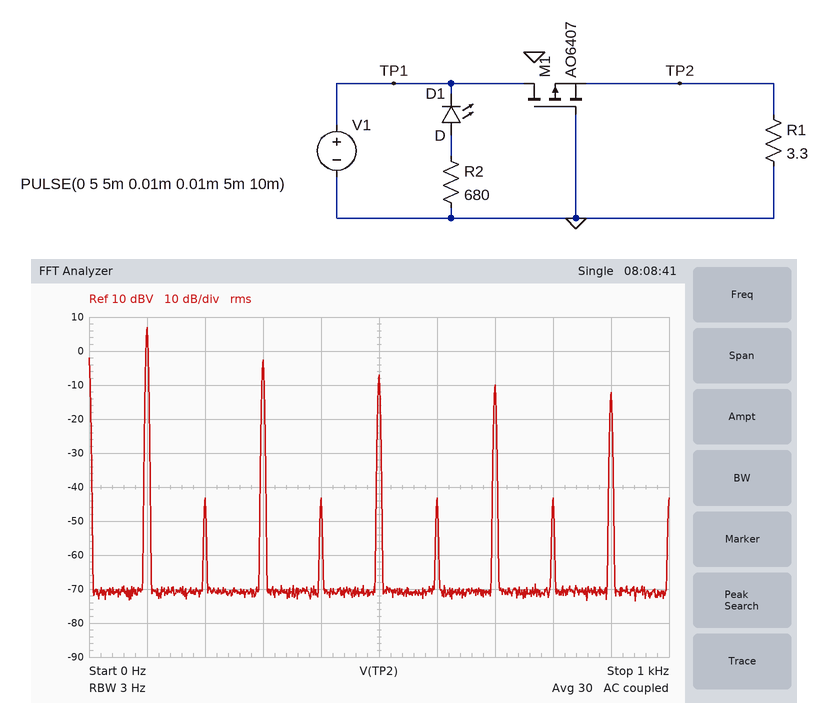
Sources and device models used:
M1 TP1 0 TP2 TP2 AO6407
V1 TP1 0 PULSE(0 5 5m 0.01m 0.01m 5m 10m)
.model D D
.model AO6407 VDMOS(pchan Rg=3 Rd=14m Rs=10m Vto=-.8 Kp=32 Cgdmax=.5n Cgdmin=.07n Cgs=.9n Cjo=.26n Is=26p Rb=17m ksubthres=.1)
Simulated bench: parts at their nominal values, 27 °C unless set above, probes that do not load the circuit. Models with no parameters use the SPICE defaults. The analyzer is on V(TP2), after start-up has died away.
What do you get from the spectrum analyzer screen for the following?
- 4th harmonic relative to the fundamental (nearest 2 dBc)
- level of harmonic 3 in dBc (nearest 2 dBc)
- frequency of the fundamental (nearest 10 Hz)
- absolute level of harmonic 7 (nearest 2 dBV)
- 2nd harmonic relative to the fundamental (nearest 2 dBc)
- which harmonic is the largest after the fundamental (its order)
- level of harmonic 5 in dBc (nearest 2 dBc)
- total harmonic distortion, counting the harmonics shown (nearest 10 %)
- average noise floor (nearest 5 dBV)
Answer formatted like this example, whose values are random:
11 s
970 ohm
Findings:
-50 dBc
-10 dBc
100 Hz
-10 dBV
-50 dBc
3
-14 dBc
40 %
-70 dBV
